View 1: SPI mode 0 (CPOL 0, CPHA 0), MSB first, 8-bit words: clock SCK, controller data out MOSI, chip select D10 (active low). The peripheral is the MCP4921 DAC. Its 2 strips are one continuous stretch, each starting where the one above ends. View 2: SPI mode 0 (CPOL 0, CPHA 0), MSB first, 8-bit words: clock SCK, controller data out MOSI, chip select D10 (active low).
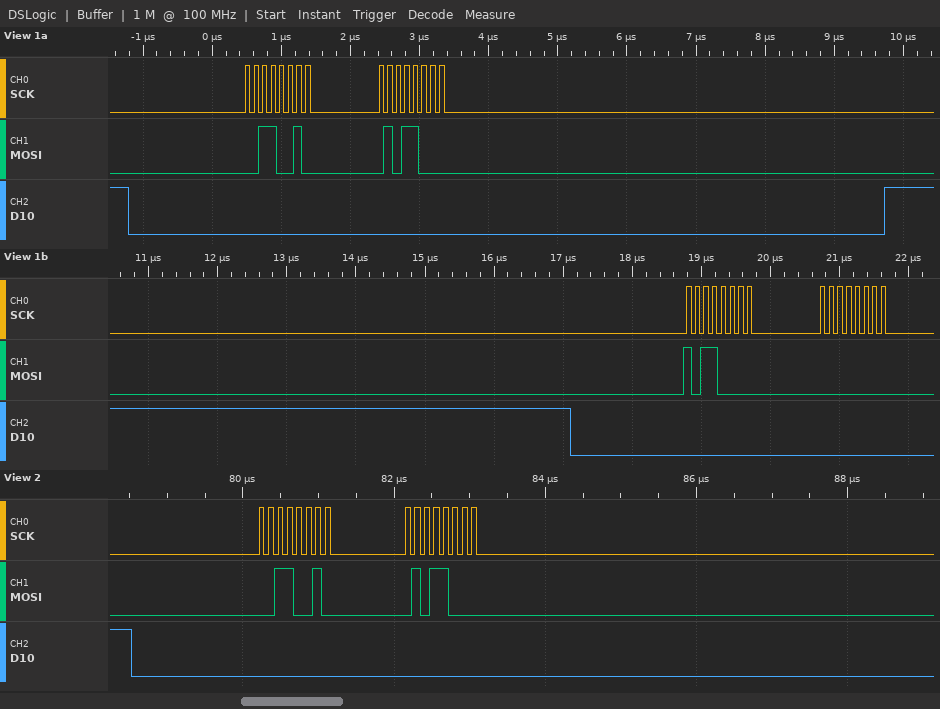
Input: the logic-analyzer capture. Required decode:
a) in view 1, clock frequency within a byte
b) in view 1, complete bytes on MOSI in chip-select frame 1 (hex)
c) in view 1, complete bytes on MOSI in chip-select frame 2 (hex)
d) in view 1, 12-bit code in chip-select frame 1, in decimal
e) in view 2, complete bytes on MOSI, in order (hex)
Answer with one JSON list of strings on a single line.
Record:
["8 MHz", "32 58", "B0 00", "600", "32 58"]
